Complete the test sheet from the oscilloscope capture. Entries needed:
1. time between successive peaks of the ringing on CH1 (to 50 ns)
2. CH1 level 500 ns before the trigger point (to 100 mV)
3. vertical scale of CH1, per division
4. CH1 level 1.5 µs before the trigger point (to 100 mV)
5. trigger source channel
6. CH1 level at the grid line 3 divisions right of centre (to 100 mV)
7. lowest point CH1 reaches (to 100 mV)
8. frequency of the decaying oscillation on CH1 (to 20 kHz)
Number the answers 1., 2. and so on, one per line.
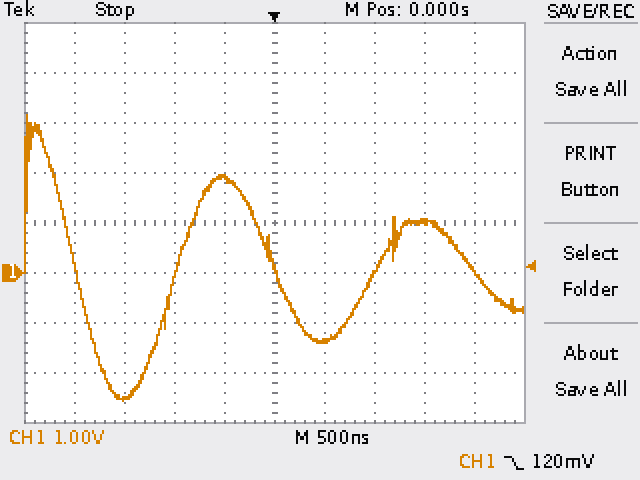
1. 1.95 µs
2. 1.9 V
3. 1 V
4. -2.5 V
5. CH1
6. 1.0 V
7. -2.6 V
8. 520 kHz
